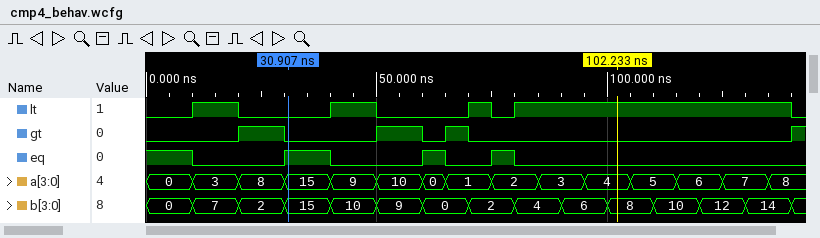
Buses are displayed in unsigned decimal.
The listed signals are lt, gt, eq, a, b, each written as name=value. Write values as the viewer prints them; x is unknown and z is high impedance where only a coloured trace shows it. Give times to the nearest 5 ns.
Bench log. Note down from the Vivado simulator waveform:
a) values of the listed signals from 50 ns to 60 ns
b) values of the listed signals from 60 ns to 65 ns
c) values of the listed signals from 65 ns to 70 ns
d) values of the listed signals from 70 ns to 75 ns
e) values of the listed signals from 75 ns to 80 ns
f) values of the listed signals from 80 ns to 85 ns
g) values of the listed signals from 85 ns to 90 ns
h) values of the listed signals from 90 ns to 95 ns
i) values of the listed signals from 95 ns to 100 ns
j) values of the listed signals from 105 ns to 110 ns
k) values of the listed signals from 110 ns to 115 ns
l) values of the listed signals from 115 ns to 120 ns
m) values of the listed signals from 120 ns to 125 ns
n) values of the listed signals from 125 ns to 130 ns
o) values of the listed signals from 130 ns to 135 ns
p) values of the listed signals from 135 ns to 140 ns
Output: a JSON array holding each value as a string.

["lt=0, gt=1, eq=0, a=10, b=9", "lt=0, gt=0, eq=1, a=0, b=0", "lt=0, gt=1, eq=0, a=1, b=0", "lt=1, gt=0, eq=0, a=1, b=2", "lt=0, gt=0, eq=1, a=2, b=2", "lt=1, gt=0, eq=0, a=2, b=4", "lt=1, gt=0, eq=0, a=3, b=4", "lt=1, gt=0, eq=0, a=3, b=6", "lt=1, gt=0, eq=0, a=4, b=6", "lt=1, gt=0, eq=0, a=5, b=8", "lt=1, gt=0, eq=0, a=5, b=10", "lt=1, gt=0, eq=0, a=6, b=10", "lt=1, gt=0, eq=0, a=6, b=12", "lt=1, gt=0, eq=0, a=7, b=12", "lt=1, gt=0, eq=0, a=7, b=14", "lt=1, gt=0, eq=0, a=8, b=14"]
